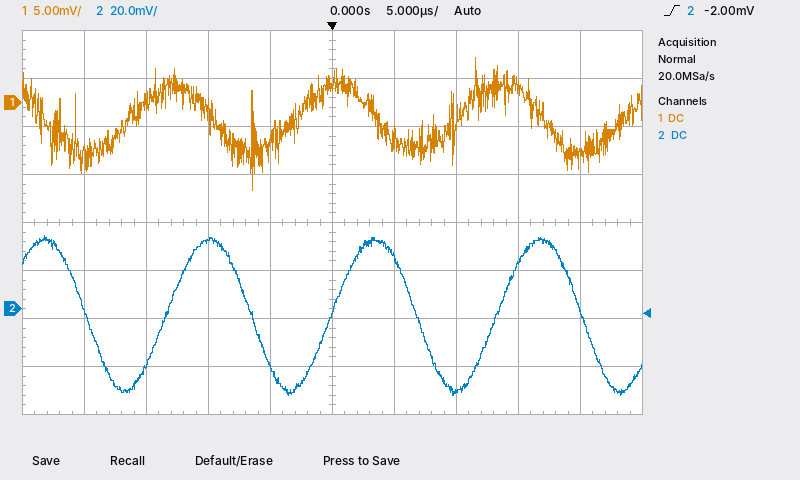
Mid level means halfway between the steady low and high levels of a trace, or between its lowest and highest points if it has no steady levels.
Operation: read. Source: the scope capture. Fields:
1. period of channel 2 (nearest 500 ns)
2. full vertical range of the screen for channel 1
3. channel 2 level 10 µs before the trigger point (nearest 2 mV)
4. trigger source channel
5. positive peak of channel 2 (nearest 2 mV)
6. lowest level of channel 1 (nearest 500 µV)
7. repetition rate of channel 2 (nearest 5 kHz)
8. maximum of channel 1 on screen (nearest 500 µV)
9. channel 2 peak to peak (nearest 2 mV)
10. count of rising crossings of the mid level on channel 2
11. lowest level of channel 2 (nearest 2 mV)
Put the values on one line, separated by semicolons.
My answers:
13.5 µs; 40 mV; 28 mV; channel 2; 30 mV; -9.0 mV; 75 kHz; 4.5 mV; 66 mV; 3; -36 mV
